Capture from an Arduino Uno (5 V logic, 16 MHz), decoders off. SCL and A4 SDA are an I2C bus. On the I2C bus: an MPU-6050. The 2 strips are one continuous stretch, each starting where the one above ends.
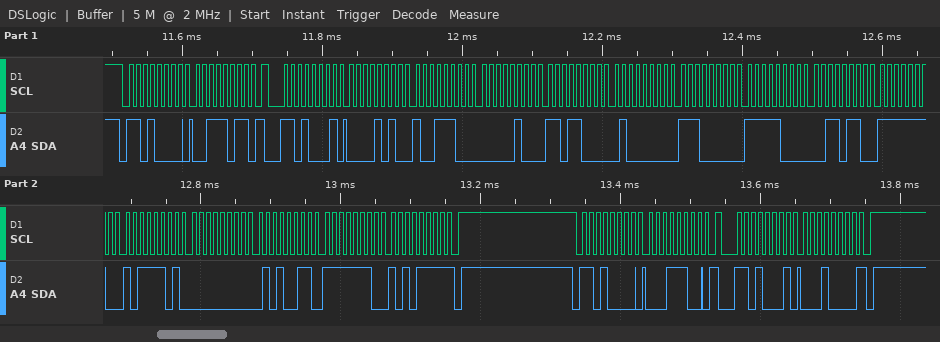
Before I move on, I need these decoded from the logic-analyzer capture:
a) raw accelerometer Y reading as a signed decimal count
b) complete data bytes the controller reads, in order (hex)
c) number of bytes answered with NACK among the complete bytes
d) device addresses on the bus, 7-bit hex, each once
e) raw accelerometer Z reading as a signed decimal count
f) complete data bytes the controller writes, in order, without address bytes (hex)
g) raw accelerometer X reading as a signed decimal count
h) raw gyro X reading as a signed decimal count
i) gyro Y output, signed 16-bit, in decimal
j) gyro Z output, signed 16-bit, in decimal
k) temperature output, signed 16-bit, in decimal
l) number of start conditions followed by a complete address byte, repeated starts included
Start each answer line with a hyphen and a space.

- 1240
- 0A 9C 04 D8 40 E0 F8 36 FE BD 00 53 FE AF 10
- 2
- 0x68
- 16608
- 3B 1C
- 2716
- -323
- 83
- -337
- -1994
- 4
